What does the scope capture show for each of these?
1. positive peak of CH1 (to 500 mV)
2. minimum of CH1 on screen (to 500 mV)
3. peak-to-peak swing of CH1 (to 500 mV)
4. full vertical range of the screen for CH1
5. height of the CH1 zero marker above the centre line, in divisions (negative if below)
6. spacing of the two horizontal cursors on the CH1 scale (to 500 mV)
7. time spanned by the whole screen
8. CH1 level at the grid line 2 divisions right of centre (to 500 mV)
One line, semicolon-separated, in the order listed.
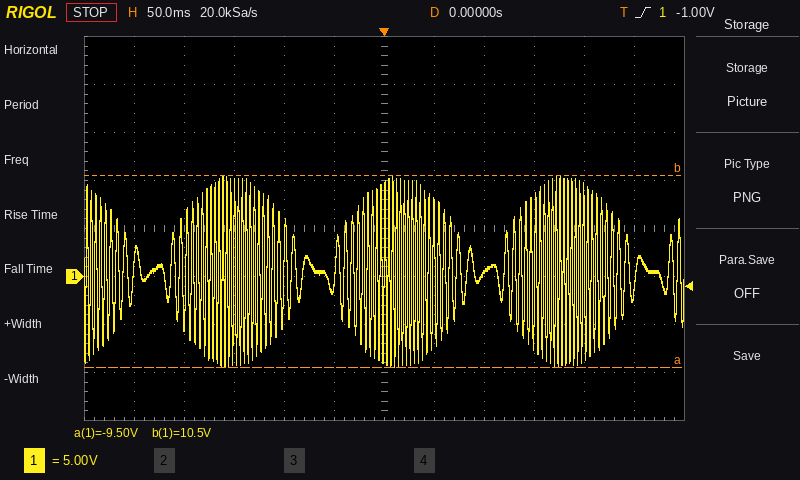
10.5 V; -9.5 V; 20.0 V; 40 V; -1.0 div; 20.0 V; 600 ms; 500 mV
